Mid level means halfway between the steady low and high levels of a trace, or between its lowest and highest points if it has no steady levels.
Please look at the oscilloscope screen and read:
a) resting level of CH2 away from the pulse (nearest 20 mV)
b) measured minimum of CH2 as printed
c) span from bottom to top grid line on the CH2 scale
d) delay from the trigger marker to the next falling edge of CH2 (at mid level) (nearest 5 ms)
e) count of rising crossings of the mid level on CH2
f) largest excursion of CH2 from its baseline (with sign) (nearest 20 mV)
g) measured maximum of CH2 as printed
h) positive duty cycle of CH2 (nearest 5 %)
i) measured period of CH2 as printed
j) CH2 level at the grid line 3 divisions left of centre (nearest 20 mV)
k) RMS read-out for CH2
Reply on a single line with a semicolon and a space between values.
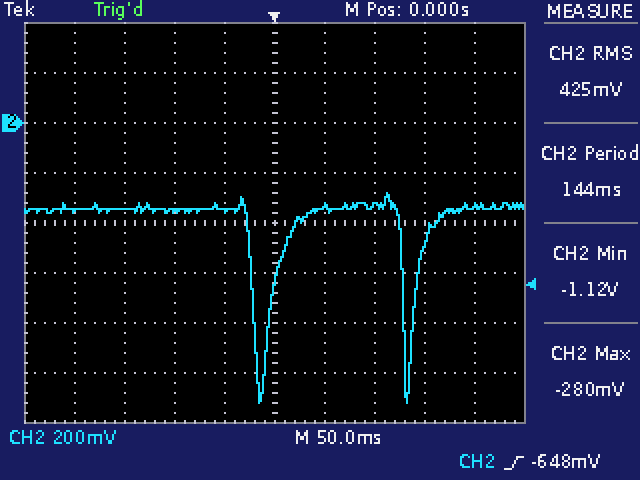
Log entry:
-340 mV; -1.12 V; 1.6 V; 130 ms; 2; -780 mV; -280 mV; 90 %; 144 ms; -340 mV; 425 mV
